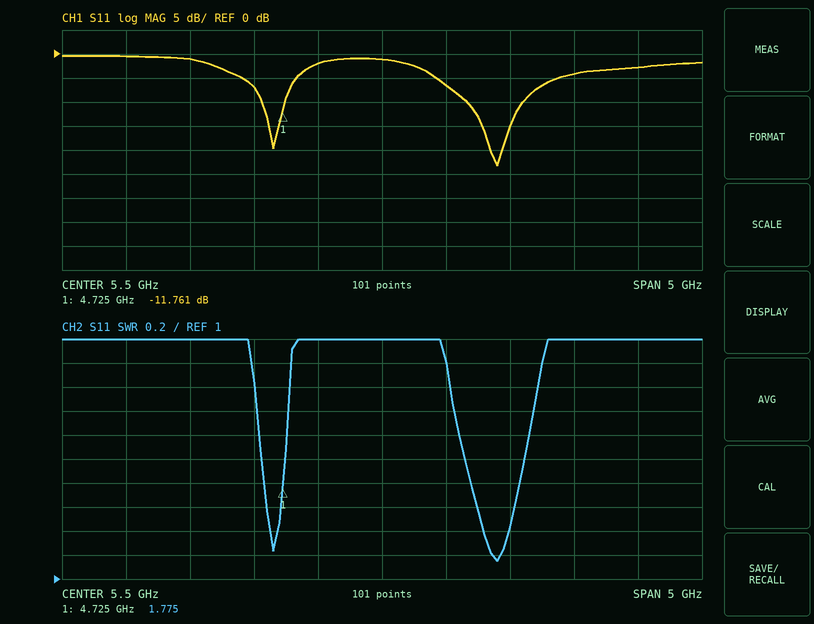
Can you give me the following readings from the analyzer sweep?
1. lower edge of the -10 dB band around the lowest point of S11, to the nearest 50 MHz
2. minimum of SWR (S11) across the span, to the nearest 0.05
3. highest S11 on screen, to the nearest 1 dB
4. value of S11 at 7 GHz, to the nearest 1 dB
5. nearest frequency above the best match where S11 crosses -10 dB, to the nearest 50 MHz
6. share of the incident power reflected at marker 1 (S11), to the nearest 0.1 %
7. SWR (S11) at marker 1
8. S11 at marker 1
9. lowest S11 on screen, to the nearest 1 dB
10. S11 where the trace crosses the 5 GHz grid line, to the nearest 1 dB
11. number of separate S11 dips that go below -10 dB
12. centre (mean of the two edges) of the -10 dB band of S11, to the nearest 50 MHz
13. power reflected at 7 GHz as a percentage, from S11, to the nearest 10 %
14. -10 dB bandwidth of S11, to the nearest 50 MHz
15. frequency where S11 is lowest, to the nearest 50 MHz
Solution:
6.15 GHz
1.15
0 dB
-4 dB
6.60 GHz
6.7 %
1.775
-11.761 dB
-23 dB
-2 dB
2
6.40 GHz
40 %
450 MHz
6.40 GHz
